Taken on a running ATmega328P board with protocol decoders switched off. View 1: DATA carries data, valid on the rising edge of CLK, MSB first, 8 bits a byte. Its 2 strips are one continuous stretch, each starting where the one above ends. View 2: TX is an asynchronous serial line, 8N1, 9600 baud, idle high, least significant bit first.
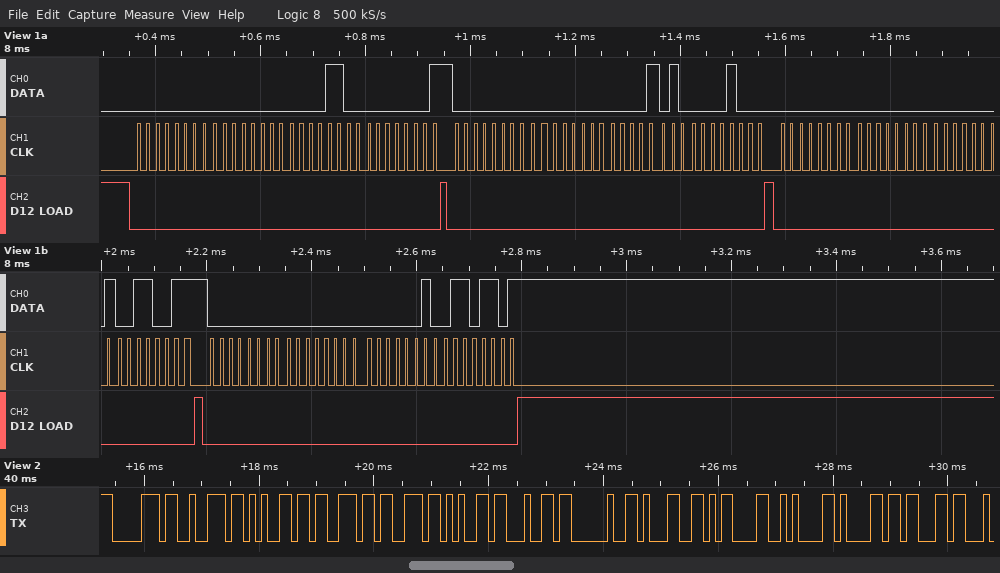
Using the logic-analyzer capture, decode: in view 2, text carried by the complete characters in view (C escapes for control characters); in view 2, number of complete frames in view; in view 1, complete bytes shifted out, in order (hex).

"pressed 1\r\nac"
13
00 00 0C 01 00 00 0A 08 00 00 01 33 00 00 02 6D
